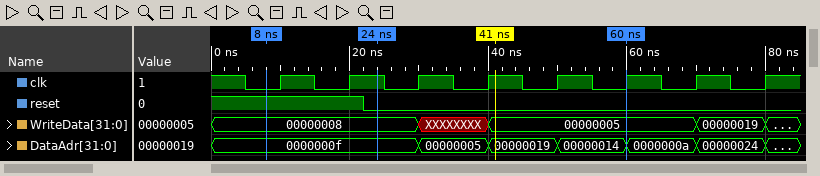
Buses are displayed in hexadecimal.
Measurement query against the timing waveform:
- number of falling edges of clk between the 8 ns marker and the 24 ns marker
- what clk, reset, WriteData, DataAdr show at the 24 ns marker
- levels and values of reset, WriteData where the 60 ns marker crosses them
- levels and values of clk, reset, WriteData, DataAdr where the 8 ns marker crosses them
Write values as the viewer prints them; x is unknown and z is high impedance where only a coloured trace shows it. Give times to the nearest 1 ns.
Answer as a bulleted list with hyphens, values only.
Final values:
- 1
- clk=1, reset=0, WriteData=00000008, DataAdr=0000000f
- reset=0, WriteData=00000005
- clk=0, reset=1, WriteData=00000008, DataAdr=0000000f
